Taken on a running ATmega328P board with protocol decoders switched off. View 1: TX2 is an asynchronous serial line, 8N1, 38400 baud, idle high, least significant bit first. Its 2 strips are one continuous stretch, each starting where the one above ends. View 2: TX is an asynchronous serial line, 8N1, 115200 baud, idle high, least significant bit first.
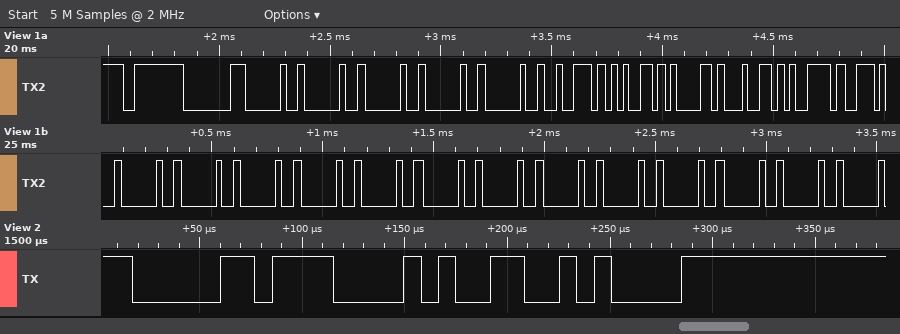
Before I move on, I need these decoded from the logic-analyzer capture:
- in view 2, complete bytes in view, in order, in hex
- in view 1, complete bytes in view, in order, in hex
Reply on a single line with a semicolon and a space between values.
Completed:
B0 28 0A; 0xFE 0x80 0x20 0x20 0x20 0x20 0x20 0x72 0x65 0x61 0x64 0x79 0x2E 0x20 0x20 0x20 0x20 0x20 0x20 0x20 0x20 0x20 0x20 0x20 0x20
